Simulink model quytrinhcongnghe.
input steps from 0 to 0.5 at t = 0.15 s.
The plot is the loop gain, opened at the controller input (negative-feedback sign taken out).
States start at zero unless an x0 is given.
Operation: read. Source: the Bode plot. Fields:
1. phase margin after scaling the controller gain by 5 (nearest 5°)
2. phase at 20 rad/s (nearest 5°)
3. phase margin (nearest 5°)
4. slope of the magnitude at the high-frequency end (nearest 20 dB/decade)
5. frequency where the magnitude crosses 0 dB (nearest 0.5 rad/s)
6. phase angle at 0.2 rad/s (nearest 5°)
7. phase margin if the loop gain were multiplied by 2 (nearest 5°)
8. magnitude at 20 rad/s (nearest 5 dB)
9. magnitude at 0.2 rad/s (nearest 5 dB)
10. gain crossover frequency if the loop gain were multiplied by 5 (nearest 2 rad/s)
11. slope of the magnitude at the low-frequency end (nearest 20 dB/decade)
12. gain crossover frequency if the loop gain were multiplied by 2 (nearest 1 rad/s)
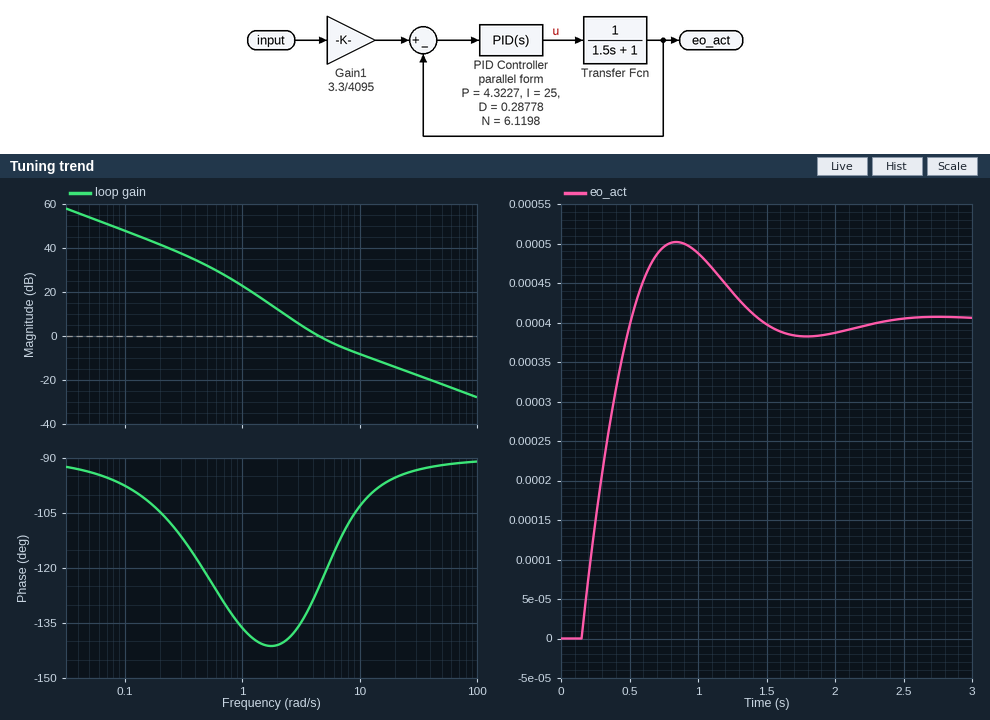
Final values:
85°
-95°
55°
-20 dB/decade
4.5 rad/s
-105°
70°
-15 dB
40 dB
20 rad/s
-20 dB/decade
8 rad/s
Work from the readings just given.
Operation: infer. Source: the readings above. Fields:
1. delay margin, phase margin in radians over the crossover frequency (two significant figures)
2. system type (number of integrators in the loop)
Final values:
0.21 s
1
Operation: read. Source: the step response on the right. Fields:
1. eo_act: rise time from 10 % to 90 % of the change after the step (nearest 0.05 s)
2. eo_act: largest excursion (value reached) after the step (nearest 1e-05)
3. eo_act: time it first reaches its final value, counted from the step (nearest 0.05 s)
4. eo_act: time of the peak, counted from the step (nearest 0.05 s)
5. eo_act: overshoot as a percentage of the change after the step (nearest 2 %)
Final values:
0.30 s
0.00050
0.35 s
0.70 s
24 %
